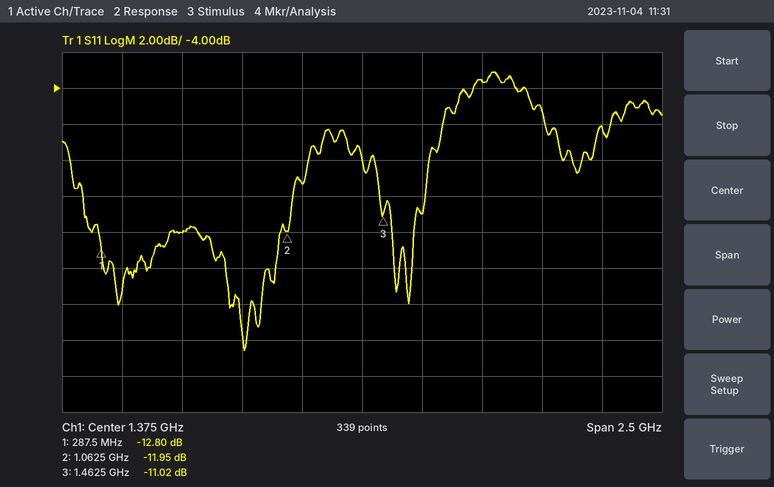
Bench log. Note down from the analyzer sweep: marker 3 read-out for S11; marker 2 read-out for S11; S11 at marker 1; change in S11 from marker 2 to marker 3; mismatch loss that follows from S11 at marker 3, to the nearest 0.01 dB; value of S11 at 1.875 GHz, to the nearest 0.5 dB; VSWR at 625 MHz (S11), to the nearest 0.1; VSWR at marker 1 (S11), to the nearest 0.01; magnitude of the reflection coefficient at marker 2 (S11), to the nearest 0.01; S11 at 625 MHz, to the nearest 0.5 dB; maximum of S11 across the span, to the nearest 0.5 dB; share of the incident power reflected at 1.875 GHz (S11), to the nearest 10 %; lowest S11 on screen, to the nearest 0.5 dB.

-11.02 dB
-11.95 dB
-12.80 dB
0.93 dB
0.36 dB
-3.5 dB
1.7
1.59
0.25
-12.0 dB
-3.0 dB
40 %
-18.5 dB
